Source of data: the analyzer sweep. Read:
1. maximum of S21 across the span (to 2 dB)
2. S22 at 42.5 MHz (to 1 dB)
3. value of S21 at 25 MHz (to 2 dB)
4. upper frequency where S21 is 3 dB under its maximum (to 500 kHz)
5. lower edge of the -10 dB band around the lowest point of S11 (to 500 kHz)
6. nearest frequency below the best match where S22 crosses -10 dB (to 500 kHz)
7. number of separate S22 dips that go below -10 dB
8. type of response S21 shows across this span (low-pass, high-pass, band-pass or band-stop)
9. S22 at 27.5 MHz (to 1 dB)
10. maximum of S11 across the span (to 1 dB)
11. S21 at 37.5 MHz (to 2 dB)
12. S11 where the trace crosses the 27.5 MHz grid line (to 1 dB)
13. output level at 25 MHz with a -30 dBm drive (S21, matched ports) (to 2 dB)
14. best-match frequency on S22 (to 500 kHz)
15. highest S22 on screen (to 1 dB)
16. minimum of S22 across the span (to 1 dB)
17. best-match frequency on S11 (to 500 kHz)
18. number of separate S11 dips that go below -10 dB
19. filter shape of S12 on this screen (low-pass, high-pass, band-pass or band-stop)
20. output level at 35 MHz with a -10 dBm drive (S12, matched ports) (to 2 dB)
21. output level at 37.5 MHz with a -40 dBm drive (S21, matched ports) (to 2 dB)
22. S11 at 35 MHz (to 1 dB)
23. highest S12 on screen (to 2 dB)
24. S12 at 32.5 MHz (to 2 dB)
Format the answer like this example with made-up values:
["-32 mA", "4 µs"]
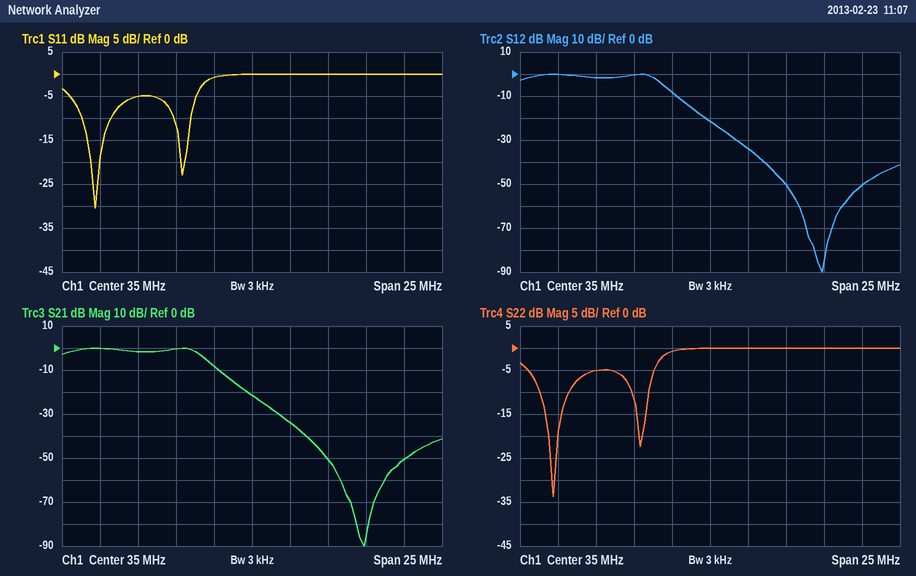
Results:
["0 dB", "0 dB", "0 dB", "31.5 MHz", "24.0 MHz", "24.0 MHz", "2", "low-pass", "-5 dB", "0 dB", "-34 dB", "-5 dB", "-30 dBm", "24.5 MHz", "0 dB", "-34 dB", "24.5 MHz", "2", "low-pass", "-32 dBm", "-74 dBm", "0 dB", "0 dB", "-8 dB"]
